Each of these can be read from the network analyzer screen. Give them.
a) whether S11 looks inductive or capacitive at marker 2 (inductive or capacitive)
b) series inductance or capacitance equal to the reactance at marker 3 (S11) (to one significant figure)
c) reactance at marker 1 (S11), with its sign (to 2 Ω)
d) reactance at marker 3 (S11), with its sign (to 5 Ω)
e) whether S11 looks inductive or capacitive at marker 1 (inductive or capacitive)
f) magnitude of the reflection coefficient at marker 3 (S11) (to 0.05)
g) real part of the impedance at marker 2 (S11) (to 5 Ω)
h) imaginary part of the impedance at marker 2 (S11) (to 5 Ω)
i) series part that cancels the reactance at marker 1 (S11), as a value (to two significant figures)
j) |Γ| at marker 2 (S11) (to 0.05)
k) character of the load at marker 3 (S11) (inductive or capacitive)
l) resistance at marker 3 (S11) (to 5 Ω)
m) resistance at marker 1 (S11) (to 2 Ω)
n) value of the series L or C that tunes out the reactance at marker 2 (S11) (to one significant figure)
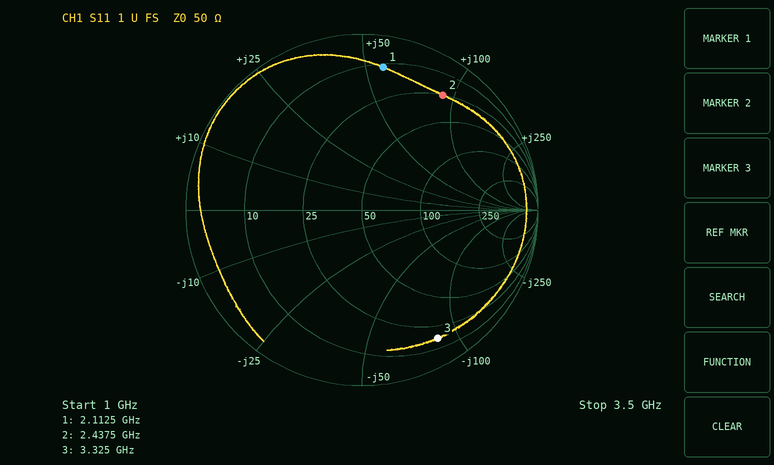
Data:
inductive
600 fF
+56 Ω
-85 Ω
inductive
0.85
25 Ω
+90 Ω
1.3 pF
0.80
capacitive
15 Ω
12 Ω
700 fF
